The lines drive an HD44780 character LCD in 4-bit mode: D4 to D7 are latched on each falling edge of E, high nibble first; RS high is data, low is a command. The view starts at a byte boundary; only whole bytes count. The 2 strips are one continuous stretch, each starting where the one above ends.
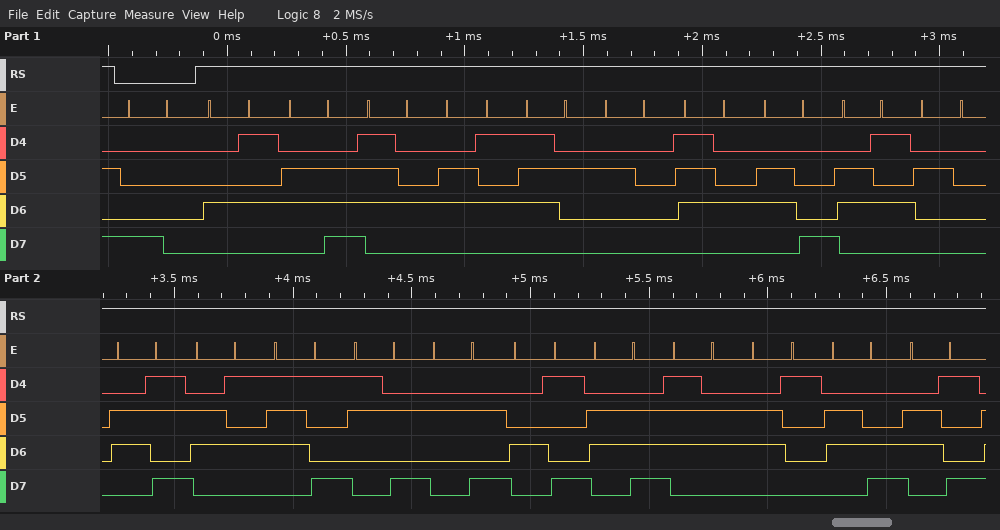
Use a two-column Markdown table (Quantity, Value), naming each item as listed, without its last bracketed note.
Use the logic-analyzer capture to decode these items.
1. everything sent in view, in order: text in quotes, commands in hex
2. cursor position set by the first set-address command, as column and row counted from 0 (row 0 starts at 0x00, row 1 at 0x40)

| Quantity | Value |
|---|---|
| everything sent in view, in order: text in quotes, commands in hex | 0x80 "Enter the key:*Invali" |
| cursor position set by the first set-address command, as column and row counted from 0 | column 0, row 0 |
